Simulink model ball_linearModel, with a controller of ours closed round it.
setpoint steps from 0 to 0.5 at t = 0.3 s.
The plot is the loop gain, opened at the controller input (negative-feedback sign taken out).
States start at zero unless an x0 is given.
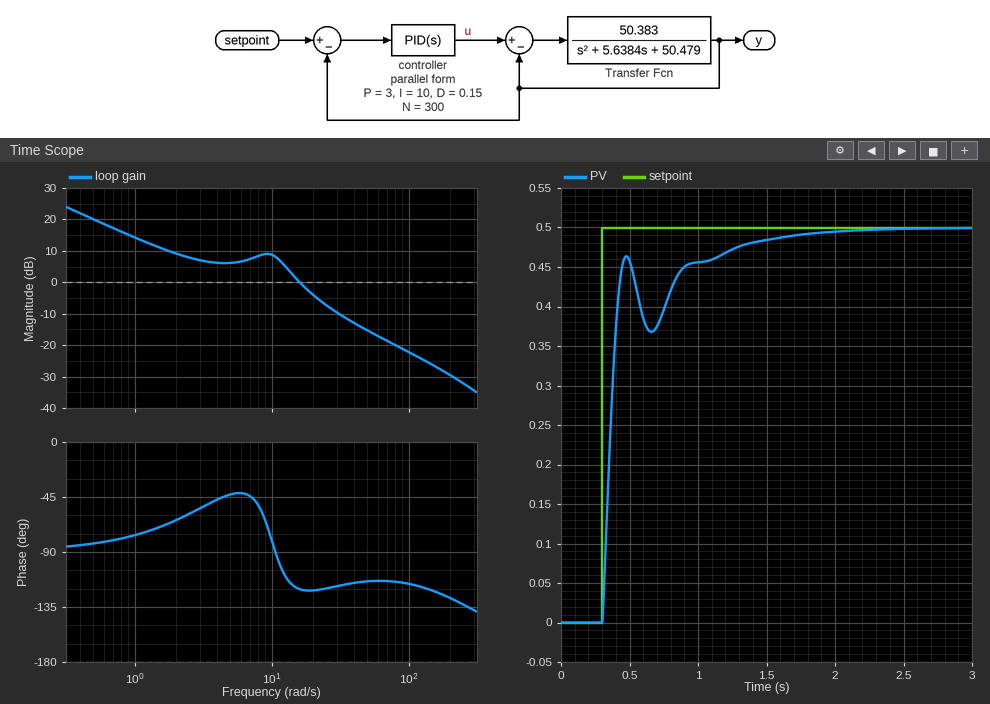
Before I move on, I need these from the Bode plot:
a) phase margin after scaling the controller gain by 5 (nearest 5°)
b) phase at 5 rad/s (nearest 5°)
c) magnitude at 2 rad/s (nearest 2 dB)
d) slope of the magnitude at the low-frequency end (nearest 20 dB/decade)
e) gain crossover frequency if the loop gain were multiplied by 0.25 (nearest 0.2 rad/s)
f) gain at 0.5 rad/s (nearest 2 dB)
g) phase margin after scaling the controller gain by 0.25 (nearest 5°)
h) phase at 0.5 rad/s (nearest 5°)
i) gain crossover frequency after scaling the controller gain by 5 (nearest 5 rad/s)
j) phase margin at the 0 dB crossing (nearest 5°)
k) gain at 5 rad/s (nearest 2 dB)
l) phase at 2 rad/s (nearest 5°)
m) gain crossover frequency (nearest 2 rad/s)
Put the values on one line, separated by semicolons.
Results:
65°; -45°; 10 dB; -20 dB/decade; 1.4 rad/s; 20 dB; 110°; -85°; 45 rad/s; 60°; 6 dB; -65°; 16 rad/s
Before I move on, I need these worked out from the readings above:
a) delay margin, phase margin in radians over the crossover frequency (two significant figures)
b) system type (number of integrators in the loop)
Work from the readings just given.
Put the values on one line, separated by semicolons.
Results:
0.065 s; 1
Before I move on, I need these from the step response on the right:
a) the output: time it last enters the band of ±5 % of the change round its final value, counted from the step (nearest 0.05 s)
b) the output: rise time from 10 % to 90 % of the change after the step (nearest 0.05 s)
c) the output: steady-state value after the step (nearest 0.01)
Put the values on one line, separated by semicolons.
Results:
1.00 s; 0.15 s; 0.50
